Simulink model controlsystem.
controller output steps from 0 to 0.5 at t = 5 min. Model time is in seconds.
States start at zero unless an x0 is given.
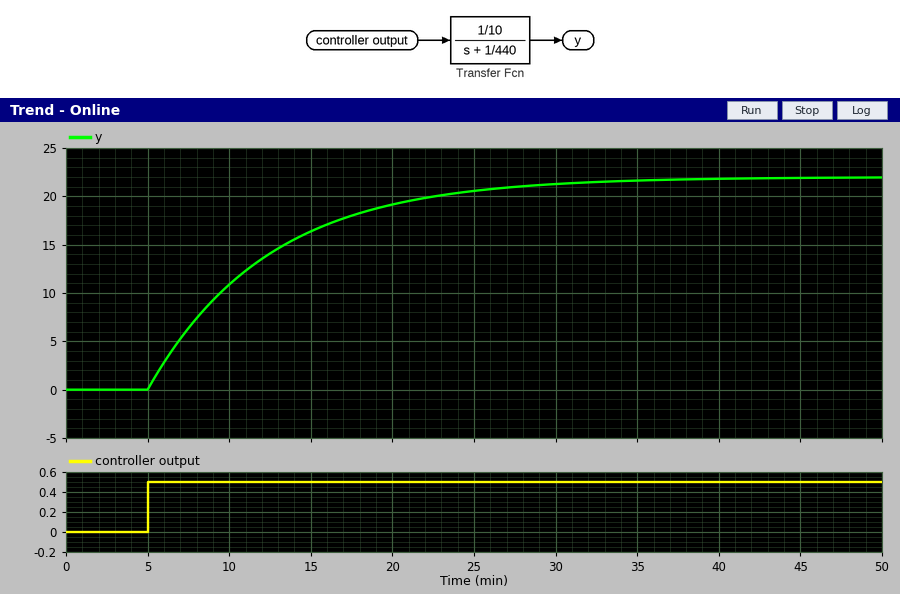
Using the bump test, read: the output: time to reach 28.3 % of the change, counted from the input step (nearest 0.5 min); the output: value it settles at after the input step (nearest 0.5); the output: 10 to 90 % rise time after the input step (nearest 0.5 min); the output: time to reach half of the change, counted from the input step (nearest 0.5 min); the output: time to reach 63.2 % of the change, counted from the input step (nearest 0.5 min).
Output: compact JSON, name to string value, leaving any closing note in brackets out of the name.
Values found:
{"the output: time to reach 28.3 % of the change, counted from the input step": "2.5 min", "the output: value it settles at after the input step": "22.0", "the output: 10 to 90 % rise time after the input step": "16.0 min", "the output: time to reach half of the change, counted from the input step": "5.0 min", "the output: time to reach 63.2 % of the change, counted from the input step": "7.5 min"}
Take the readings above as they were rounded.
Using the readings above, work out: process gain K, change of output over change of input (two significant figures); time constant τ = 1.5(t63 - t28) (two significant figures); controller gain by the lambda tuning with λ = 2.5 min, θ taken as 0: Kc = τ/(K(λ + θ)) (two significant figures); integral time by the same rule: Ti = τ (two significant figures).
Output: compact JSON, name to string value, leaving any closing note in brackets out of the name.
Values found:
{"process gain K, change of output over change of input": "44", "time constant τ = 1.5(t63 - t28)": "7.5 min", "controller gain by the lambda tuning with λ = 2.5 min, θ taken as 0: Kc = τ/(K(λ + θ))": "0.068", "integral time by the same rule: Ti = τ": "7.5 min"}
